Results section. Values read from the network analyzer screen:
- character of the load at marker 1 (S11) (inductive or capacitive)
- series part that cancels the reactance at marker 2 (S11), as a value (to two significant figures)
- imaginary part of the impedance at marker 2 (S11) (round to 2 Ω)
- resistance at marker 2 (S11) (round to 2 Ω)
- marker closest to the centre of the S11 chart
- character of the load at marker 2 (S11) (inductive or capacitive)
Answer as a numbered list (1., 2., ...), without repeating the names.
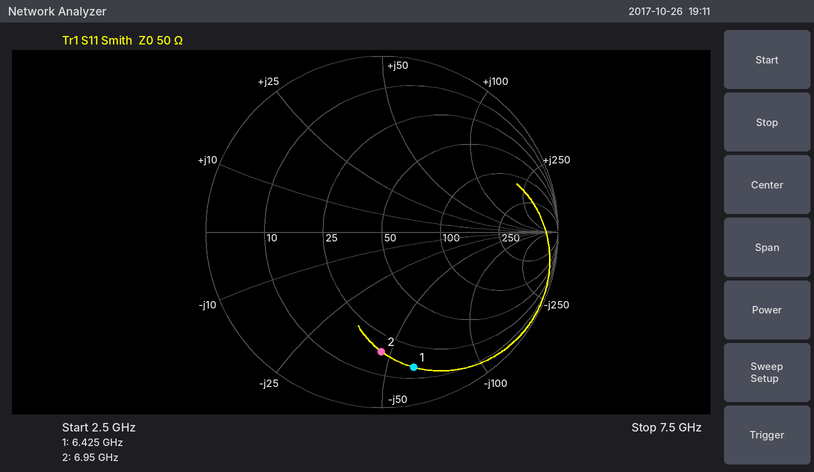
1. capacitive
2. 1.1 nH
3. -46 Ω
4. 18 Ω
5. marker 2
6. capacitive
